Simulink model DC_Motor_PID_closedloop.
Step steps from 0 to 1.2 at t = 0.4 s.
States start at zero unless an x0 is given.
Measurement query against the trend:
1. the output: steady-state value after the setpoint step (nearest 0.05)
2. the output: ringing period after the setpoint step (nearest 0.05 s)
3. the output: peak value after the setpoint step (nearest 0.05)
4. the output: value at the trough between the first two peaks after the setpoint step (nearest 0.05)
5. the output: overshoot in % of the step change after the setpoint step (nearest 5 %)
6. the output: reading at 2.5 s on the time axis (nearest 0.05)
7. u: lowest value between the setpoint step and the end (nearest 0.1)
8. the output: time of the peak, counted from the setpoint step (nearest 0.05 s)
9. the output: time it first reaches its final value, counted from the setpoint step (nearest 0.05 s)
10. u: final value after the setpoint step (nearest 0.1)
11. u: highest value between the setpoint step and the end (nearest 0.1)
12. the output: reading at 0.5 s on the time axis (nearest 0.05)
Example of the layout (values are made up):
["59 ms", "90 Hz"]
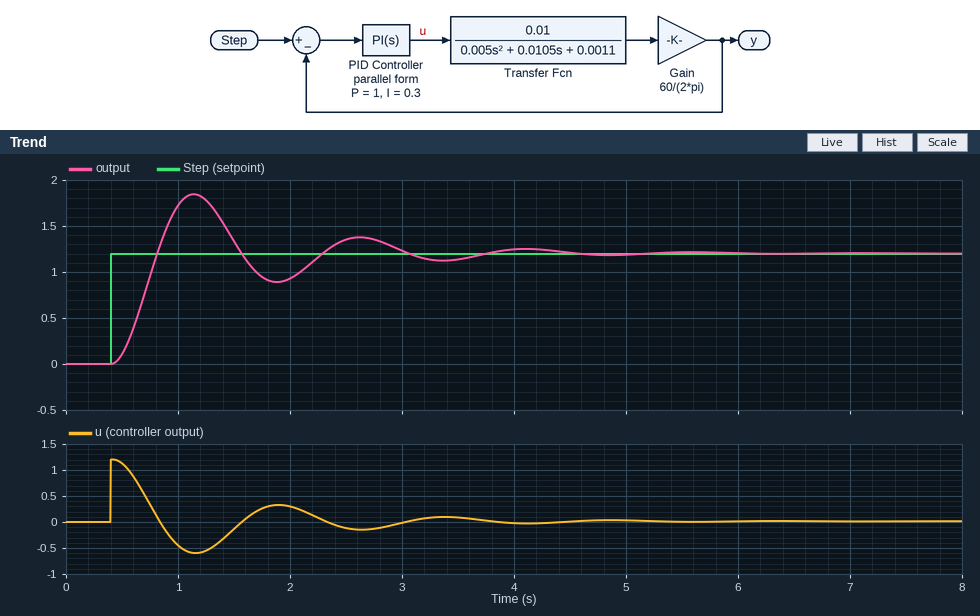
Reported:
["1.20", "1.50 s", "1.85", "0.90", "55 %", "1.35", "-0.6", "0.75 s", "0.40 s", "0.0", "1.2", "0.10"]
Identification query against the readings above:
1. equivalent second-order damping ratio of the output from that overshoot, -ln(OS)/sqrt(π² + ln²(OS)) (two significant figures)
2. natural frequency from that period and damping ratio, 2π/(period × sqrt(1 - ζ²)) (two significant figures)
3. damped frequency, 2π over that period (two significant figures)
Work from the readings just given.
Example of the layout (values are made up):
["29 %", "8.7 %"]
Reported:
["0.19", "4.3 rad/s", "4.2 rad/s"]
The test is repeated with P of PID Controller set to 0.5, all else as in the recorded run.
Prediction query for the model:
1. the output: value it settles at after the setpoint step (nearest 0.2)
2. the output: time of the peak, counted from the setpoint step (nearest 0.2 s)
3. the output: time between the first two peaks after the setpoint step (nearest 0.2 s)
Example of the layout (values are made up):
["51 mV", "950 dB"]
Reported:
["1.2", "1.0 s", "2.2 s"]
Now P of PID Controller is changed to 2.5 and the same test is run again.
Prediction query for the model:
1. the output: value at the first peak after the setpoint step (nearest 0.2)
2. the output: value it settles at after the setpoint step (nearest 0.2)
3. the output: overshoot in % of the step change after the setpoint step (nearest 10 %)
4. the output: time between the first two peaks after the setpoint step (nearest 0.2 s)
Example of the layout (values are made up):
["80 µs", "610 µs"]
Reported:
["2.0", "1.2", "60 %", "1.0 s"]
